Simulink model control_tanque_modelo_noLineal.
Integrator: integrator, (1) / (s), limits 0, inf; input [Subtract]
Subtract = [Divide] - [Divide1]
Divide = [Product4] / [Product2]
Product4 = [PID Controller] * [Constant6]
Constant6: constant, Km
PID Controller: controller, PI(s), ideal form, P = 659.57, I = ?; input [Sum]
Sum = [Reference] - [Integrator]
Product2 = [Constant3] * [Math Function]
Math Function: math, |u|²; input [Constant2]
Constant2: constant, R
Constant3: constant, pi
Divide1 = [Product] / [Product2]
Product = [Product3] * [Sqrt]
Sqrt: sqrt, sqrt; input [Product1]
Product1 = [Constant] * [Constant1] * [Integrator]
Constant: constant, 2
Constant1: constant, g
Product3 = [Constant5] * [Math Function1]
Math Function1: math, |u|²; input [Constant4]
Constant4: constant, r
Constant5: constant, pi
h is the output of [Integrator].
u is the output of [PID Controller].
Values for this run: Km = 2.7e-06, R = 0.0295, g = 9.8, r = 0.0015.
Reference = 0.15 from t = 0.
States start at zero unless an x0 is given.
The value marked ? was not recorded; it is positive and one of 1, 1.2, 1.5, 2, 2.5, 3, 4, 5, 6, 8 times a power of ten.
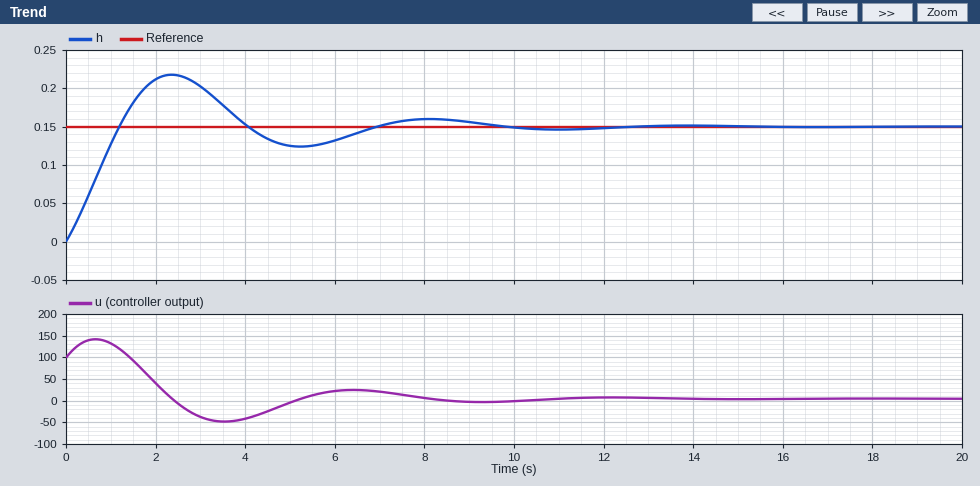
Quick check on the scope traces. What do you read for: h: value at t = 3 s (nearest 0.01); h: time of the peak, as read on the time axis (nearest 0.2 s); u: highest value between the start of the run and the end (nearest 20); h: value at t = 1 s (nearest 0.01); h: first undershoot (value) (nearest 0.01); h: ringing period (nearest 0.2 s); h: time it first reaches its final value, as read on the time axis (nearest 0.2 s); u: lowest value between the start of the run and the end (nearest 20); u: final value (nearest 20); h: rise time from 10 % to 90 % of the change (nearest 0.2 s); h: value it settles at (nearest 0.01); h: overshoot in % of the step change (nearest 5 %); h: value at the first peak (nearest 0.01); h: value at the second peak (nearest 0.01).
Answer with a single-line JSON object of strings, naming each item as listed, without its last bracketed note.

{"h: value at t = 3 s": "0.20", "h: time of the peak, as read on the time axis": "2.4 s", "u: highest value between the start of the run and the end": "140", "h: value at t = 1 s": "0.13", "h: first undershoot (value)": "0.12", "h: ringing period": "5.8 s", "h: time it first reaches its final value, as read on the time axis": "1.2 s", "u: lowest value between the start of the run and the end": "-40", "u: final value": "0", "h: rise time from 10 % to 90 % of the change": "1.0 s", "h: value it settles at": "0.15", "h: overshoot in % of the step change": "45 %", "h: value at the first peak": "0.22", "h: value at the second peak": "0.16"}
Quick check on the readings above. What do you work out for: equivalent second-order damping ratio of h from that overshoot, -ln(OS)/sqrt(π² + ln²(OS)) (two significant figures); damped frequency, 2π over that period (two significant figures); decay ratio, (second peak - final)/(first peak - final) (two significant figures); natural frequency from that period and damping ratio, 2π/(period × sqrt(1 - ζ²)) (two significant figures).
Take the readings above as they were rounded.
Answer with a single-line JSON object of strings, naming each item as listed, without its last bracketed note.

{"equivalent second-order damping ratio of h from that overshoot, -ln(OS)/sqrt(π² + ln²(OS))": "0.25", "damped frequency, 2π over that period": "1.1 rad/s", "decay ratio, (second peak - final)/(first peak - final)": "0.14", "natural frequency from that period and damping ratio, 2π/(period × sqrt(1 - ζ²))": "1.1 rad/s"}
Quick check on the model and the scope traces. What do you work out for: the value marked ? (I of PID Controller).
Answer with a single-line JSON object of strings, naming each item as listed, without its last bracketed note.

{"the value marked ?": "2"}
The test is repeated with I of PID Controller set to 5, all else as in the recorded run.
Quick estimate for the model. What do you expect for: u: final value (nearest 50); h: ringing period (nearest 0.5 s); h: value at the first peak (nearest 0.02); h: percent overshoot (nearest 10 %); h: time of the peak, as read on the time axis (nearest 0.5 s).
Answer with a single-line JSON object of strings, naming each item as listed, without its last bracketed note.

{"u: final value": "0", "h: ringing period": "3.5 s", "h: value at the first peak": "0.24", "h: percent overshoot": "60 %", "h: time of the peak, as read on the time axis": "1.5 s"}
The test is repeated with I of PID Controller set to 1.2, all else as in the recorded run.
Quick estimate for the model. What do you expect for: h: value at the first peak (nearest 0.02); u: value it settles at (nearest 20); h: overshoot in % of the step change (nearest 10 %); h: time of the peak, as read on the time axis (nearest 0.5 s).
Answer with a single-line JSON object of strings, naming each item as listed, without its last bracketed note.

{"h: value at the first peak": "0.20", "u: value it settles at": "0", "h: overshoot in % of the step change": "40 %", "h: time of the peak, as read on the time axis": "3.0 s"}
